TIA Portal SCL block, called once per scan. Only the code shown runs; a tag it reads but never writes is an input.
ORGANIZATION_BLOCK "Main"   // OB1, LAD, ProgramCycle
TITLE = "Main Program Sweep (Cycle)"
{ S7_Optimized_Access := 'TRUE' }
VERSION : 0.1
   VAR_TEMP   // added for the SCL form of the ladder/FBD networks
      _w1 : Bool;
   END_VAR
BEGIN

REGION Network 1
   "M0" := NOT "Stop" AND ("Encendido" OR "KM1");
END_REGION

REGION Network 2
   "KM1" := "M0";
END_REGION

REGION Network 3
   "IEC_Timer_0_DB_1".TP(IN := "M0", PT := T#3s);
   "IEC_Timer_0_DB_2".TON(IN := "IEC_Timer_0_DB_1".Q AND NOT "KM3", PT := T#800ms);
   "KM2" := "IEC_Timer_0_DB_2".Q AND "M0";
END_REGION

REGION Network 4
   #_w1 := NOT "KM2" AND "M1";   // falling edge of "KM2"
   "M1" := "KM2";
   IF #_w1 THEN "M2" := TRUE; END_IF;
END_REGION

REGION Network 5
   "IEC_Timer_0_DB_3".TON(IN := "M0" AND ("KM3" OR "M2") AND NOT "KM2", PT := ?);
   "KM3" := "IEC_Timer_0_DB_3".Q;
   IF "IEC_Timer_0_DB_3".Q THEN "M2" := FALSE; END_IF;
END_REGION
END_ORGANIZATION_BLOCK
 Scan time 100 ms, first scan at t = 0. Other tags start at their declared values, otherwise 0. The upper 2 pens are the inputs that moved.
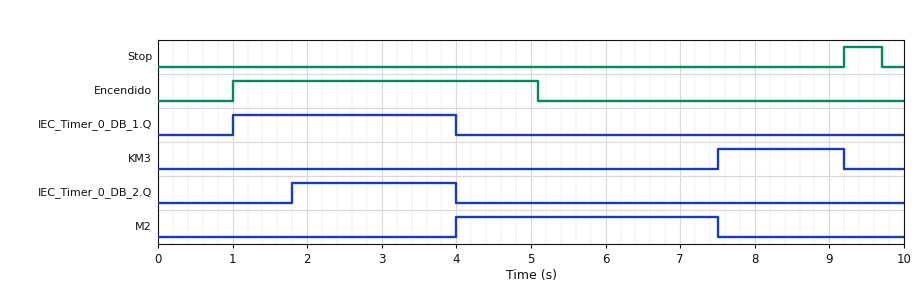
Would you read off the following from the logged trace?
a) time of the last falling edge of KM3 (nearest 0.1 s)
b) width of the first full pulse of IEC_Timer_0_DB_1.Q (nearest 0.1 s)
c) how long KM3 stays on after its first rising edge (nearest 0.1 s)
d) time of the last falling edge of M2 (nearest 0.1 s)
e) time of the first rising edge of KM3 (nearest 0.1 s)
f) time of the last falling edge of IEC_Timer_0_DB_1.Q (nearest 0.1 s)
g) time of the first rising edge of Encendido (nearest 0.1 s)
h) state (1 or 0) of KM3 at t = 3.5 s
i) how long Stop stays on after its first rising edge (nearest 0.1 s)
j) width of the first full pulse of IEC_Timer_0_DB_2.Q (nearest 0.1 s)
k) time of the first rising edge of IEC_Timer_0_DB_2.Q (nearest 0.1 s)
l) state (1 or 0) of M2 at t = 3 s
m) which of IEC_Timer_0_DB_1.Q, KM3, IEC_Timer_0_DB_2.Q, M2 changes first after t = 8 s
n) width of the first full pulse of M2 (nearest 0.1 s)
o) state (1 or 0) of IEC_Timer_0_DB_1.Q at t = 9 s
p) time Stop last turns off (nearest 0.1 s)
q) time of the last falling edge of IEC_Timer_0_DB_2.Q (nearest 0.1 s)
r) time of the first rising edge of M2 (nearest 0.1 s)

9.2 s
3.0 s
1.7 s
7.5 s
7.5 s
4.0 s
1.0 s
0
0.5 s
2.2 s
1.8 s
0
KM3
3.5 s
0
9.7 s
4.0 s
4.0 s
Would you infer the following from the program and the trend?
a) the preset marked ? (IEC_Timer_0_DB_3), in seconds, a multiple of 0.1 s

3.5 s
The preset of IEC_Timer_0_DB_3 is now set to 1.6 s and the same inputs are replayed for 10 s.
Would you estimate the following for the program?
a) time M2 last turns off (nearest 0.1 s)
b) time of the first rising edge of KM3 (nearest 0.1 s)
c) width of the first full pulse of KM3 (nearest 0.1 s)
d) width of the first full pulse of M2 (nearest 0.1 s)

5.6 s
5.6 s
3.6 s
1.6 s
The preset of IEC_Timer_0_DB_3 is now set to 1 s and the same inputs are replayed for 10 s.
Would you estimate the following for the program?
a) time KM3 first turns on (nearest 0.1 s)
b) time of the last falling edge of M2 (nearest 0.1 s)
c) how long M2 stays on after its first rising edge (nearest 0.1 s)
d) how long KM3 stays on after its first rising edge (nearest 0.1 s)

5.0 s
5.0 s
1.0 s
4.2 s
